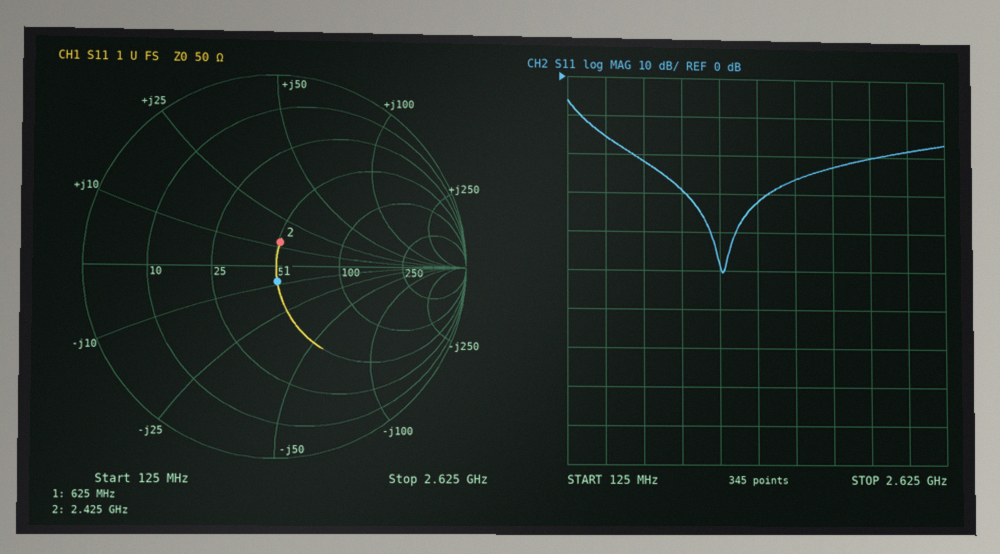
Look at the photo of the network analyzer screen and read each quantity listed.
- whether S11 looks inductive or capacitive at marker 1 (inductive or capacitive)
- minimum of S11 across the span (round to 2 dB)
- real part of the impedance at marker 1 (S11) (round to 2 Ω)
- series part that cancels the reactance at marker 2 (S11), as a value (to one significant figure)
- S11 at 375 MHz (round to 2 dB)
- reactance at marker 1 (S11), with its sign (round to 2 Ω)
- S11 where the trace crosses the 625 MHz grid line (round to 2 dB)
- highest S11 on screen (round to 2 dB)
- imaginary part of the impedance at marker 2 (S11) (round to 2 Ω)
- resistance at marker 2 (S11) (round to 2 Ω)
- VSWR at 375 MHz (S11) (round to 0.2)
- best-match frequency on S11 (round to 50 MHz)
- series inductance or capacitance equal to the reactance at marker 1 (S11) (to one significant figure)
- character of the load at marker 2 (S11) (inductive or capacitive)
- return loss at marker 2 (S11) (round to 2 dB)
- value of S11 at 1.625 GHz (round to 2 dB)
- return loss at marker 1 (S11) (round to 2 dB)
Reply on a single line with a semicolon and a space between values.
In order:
capacitive; -50 dB; 50 Ω; 5 pF; -16 dB; -8 Ω; -22 dB; -6 dB; +12 Ω; 50 Ω; 1.4; 1.15 GHz; 30 pF; inductive; 18 dB; -26 dB; 22 dB
